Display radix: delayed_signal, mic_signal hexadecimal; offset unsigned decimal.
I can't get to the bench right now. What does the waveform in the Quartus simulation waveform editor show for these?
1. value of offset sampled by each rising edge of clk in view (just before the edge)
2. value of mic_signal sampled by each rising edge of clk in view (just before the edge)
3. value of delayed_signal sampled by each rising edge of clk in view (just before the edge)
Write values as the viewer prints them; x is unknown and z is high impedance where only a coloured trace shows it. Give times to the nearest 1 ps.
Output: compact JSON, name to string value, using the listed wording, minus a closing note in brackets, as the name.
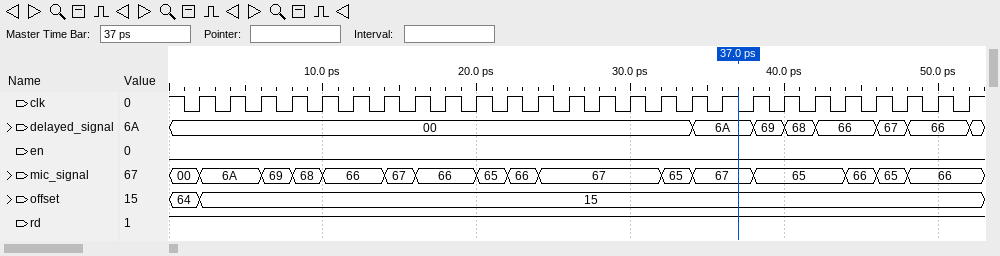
{"value of offset sampled by each rising edge of clk in view": "64, 15, 15, 15, 15, 15, 15, 15, 15, 15, 15, 15, 15, 15, 15, 15, 15, 15, 15, 15, 15, 15, 15, 15, 15, 15", "value of mic_signal sampled by each rising edge of clk in view": "00, 6A, 6A, 69, 68, 66, 66, 67, 66, 66, 65, 66, 67, 67, 67, 67, 65, 67, 67, 65, 65, 65, 66, 65, 66, 66", "value of delayed_signal sampled by each rising edge of clk in view": "00, 00, 00, 00, 00, 00, 00, 00, 00, 00, 00, 00, 00, 00, 00, 00, 00, 6A, 6A, 69, 68, 66, 66, 67, 66, 66"}
